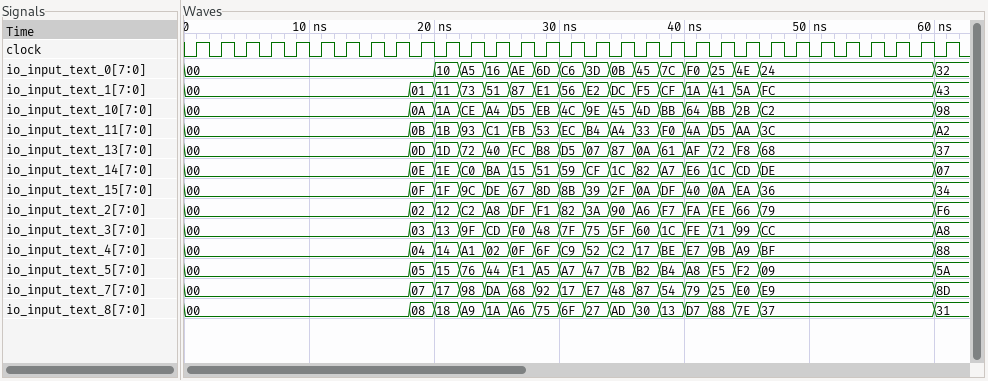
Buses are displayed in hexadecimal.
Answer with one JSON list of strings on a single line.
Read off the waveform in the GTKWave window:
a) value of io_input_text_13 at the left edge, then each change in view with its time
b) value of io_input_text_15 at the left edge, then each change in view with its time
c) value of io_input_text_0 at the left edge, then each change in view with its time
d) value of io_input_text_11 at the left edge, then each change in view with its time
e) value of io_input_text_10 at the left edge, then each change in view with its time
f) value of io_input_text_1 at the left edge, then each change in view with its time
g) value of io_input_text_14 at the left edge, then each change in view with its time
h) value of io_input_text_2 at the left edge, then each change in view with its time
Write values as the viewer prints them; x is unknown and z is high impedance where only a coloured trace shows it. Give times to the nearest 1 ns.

["00, 0D at 18 ns, 1D at 20 ns, 72 at 22 ns, 40 at 24 ns, FC at 26 ns, B8 at 28 ns, D5 at 30 ns, 07 at 32 ns, 87 at 34 ns, 0A at 36 ns, 61 at 38 ns, AF at 40 ns, 72 at 42 ns, F8 at 44 ns, 68 at 46 ns, 37 at 60 ns", "00, 0F at 18 ns, 1F at 20 ns, 9C at 22 ns, DE at 24 ns, 67 at 26 ns, 8D at 28 ns, 8B at 30 ns, 39 at 32 ns, 2F at 34 ns, 0A at 36 ns, DF at 38 ns, 40 at 40 ns, 0A at 42 ns, EA at 44 ns, 36 at 46 ns, 34 at 60 ns", "00, 10 at 20 ns, A5 at 22 ns, 16 at 24 ns, AE at 26 ns, 6D at 28 ns, C6 at 30 ns, 3D at 32 ns, 0B at 34 ns, 45 at 36 ns, 7C at 38 ns, F0 at 40 ns, 25 at 42 ns, 4E at 44 ns, 24 at 46 ns, 32 at 60 ns", "00, 0B at 18 ns, 1B at 20 ns, 93 at 22 ns, C1 at 24 ns, FB at 26 ns, 53 at 28 ns, EC at 30 ns, B4 at 32 ns, A4 at 34 ns, 33 at 36 ns, F0 at 38 ns, 4A at 40 ns, D5 at 42 ns, AA at 44 ns, 3C at 46 ns, A2 at 60 ns", "00, 0A at 18 ns, 1A at 20 ns, CE at 22 ns, A4 at 24 ns, D5 at 26 ns, EB at 28 ns, 4C at 30 ns, 9E at 32 ns, 45 at 34 ns, 4D at 36 ns, BB at 38 ns, 64 at 40 ns, BB at 42 ns, 2B at 44 ns, C2 at 46 ns, 98 at 60 ns", "00, 01 at 18 ns, 11 at 20 ns, 73 at 22 ns, 51 at 24 ns, 87 at 26 ns, E1 at 28 ns, 56 at 30 ns, E2 at 32 ns, DC at 34 ns, F5 at 36 ns, CF at 38 ns, 1A at 40 ns, 41 at 42 ns, 5A at 44 ns, FC at 46 ns, 43 at 60 ns", "00, 0E at 18 ns, 1E at 20 ns, C0 at 22 ns, BA at 24 ns, 15 at 26 ns, 51 at 28 ns, 59 at 30 ns, CF at 32 ns, 1C at 34 ns, 82 at 36 ns, A7 at 38 ns, E6 at 40 ns, 1C at 42 ns, CD at 44 ns, DE at 46 ns, 07 at 60 ns", "00, 02 at 18 ns, 12 at 20 ns, C2 at 22 ns, A8 at 24 ns, DF at 26 ns, F1 at 28 ns, 82 at 30 ns, 3A at 32 ns, 90 at 34 ns, A6 at 36 ns, F7 at 38 ns, FA at 40 ns, FE at 42 ns, 66 at 44 ns, 79 at 46 ns, F6 at 60 ns"]
